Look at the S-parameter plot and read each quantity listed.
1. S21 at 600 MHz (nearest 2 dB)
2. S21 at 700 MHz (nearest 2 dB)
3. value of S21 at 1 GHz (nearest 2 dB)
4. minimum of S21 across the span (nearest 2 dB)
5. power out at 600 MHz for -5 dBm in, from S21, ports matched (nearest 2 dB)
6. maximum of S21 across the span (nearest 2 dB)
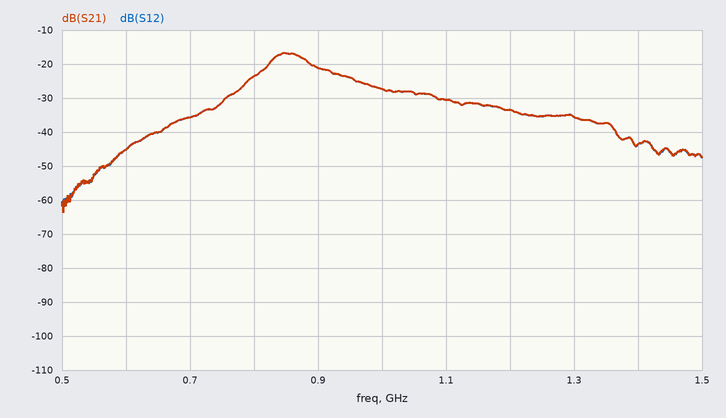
-46 dB
-36 dB
-28 dB
-64 dB
-50 dBm
-16 dB
